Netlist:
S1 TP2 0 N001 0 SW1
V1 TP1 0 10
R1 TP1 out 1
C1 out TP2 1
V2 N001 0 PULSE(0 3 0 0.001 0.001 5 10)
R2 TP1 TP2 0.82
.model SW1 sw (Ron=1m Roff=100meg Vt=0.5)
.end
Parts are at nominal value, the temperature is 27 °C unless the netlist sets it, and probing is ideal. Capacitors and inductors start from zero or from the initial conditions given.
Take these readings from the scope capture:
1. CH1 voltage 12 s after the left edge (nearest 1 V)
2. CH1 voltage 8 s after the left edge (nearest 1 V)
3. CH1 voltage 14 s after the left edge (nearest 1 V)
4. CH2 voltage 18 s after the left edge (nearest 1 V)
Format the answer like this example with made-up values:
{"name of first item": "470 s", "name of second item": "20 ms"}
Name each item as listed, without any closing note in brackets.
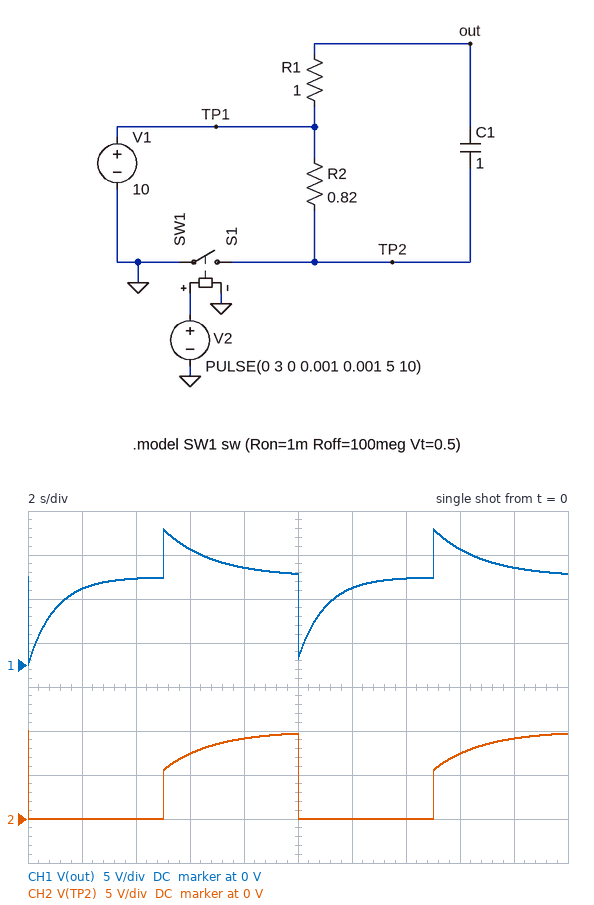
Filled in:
{"CH1 voltage 12 s after the left edge": "9 V", "CH1 voltage 8 s after the left edge": "11 V", "CH1 voltage 14 s after the left edge": "10 V", "CH2 voltage 18 s after the left edge": "9 V"}
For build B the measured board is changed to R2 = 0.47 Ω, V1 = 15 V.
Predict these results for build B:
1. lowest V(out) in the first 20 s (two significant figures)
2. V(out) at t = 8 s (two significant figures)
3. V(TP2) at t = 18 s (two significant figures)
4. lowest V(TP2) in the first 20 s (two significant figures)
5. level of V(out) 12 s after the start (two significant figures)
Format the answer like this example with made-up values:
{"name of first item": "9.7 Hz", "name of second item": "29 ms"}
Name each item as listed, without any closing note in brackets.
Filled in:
{"lowest V(out) in the first 20 s": "47 mV", "V(out) at t = 8 s": "16 V", "V(TP2) at t = 18 s": "14 V", "lowest V(TP2) in the first 20 s": "32 mV", "level of V(out) 12 s after the start": "13 V"}
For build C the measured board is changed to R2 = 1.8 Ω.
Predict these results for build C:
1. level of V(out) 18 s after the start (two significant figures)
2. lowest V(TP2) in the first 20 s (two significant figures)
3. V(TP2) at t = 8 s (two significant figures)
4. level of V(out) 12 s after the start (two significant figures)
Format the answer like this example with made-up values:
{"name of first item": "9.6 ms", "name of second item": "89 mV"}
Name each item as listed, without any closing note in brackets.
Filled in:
{"level of V(out) 18 s after the start": "11 V", "lowest V(TP2) in the first 20 s": "5.6 mV", "V(TP2) at t = 8 s": "7.8 V", "level of V(out) 12 s after the start": "8.9 V"}
